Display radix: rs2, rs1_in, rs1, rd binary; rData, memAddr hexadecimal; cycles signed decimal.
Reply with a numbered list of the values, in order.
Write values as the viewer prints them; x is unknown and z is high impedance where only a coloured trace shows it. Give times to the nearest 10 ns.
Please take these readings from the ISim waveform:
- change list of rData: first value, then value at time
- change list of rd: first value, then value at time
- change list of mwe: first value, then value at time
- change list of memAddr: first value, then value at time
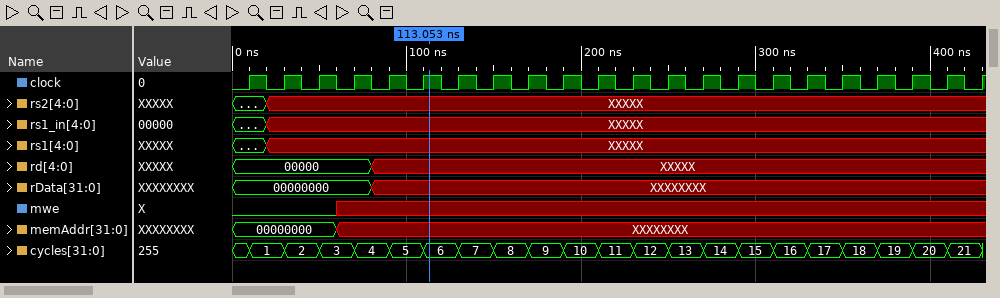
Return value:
1. 00000000, XXXXXXXX at 80 ns
2. 00000, XXXXX at 80 ns
3. 0, x at 60 ns
4. 00000000, XXXXXXXX at 60 ns
